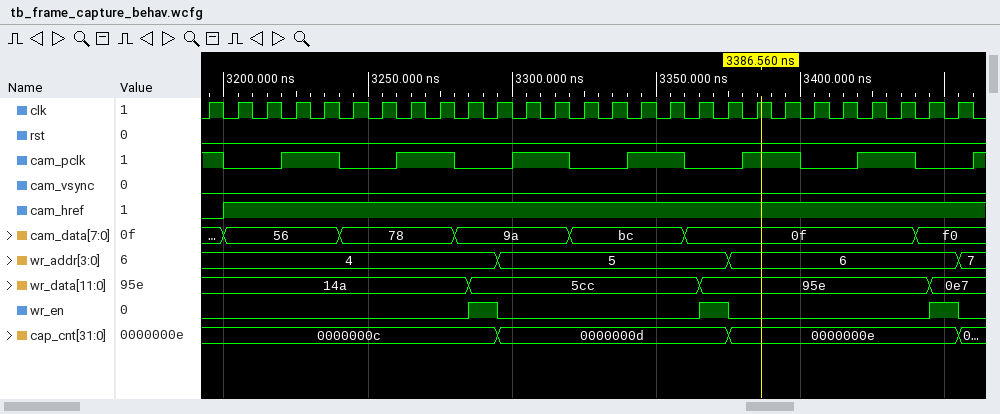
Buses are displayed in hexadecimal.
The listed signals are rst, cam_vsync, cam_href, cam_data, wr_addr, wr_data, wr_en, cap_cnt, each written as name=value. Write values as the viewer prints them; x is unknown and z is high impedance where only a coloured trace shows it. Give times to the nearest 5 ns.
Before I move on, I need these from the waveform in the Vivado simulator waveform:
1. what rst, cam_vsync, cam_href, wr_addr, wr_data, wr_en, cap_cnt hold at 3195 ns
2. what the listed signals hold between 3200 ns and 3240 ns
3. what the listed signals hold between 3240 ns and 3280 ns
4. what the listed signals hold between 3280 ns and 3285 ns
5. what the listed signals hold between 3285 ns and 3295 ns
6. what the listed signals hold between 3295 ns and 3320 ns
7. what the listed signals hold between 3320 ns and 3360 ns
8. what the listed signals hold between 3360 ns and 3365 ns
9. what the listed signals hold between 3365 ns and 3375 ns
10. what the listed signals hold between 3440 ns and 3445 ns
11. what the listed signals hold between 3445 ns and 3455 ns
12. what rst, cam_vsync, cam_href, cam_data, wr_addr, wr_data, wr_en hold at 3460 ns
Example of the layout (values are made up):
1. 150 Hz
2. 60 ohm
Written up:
1. rst=0, cam_vsync=0, cam_href=0, wr_addr=4, wr_data=14a, wr_en=0, cap_cnt=0000000c
2. rst=0, cam_vsync=0, cam_href=1, cam_data=56, wr_addr=4, wr_data=14a, wr_en=0, cap_cnt=0000000c
3. rst=0, cam_vsync=0, cam_href=1, cam_data=78, wr_addr=4, wr_data=14a, wr_en=0, cap_cnt=0000000c
4. rst=0, cam_vsync=0, cam_href=1, cam_data=9a, wr_addr=4, wr_data=14a, wr_en=0, cap_cnt=0000000c
5. rst=0, cam_vsync=0, cam_href=1, cam_data=9a, wr_addr=4, wr_data=5cc, wr_en=1, cap_cnt=0000000c
6. rst=0, cam_vsync=0, cam_href=1, cam_data=9a, wr_addr=5, wr_data=5cc, wr_en=0, cap_cnt=0000000d
7. rst=0, cam_vsync=0, cam_href=1, cam_data=bc, wr_addr=5, wr_data=5cc, wr_en=0, cap_cnt=0000000d
8. rst=0, cam_vsync=0, cam_href=1, cam_data=0f, wr_addr=5, wr_data=5cc, wr_en=0, cap_cnt=0000000d
9. rst=0, cam_vsync=0, cam_href=1, cam_data=0f, wr_addr=5, wr_data=95e, wr_en=1, cap_cnt=0000000d
10. rst=0, cam_vsync=0, cam_href=1, cam_data=f0, wr_addr=6, wr_data=95e, wr_en=0, cap_cnt=0000000e
11. rst=0, cam_vsync=0, cam_href=1, cam_data=f0, wr_addr=6, wr_data=0e7, wr_en=1, cap_cnt=0000000e
12. rst=0, cam_vsync=0, cam_href=1, cam_data=f0, wr_addr=7, wr_data=0e7, wr_en=0
